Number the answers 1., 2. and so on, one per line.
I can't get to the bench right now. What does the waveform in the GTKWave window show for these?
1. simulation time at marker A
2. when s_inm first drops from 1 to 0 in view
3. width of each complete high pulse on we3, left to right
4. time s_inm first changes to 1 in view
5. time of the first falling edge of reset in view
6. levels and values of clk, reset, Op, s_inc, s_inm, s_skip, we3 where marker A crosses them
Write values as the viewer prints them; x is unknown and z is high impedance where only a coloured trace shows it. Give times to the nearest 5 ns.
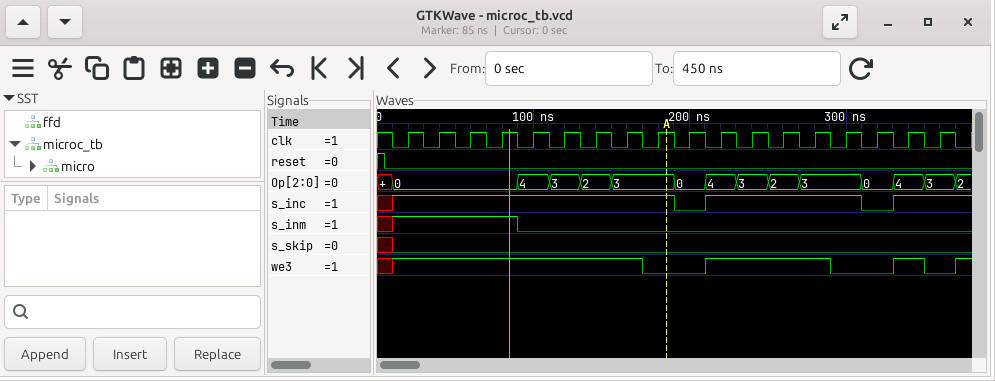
1. 185 ns
2. 90 ns
3. 80 ns, 20 ns
4. 10 ns
5. 5 ns
6. clk=1, reset=0, Op=3, s_inc=1, s_inm=0, s_skip=0, we3=0
